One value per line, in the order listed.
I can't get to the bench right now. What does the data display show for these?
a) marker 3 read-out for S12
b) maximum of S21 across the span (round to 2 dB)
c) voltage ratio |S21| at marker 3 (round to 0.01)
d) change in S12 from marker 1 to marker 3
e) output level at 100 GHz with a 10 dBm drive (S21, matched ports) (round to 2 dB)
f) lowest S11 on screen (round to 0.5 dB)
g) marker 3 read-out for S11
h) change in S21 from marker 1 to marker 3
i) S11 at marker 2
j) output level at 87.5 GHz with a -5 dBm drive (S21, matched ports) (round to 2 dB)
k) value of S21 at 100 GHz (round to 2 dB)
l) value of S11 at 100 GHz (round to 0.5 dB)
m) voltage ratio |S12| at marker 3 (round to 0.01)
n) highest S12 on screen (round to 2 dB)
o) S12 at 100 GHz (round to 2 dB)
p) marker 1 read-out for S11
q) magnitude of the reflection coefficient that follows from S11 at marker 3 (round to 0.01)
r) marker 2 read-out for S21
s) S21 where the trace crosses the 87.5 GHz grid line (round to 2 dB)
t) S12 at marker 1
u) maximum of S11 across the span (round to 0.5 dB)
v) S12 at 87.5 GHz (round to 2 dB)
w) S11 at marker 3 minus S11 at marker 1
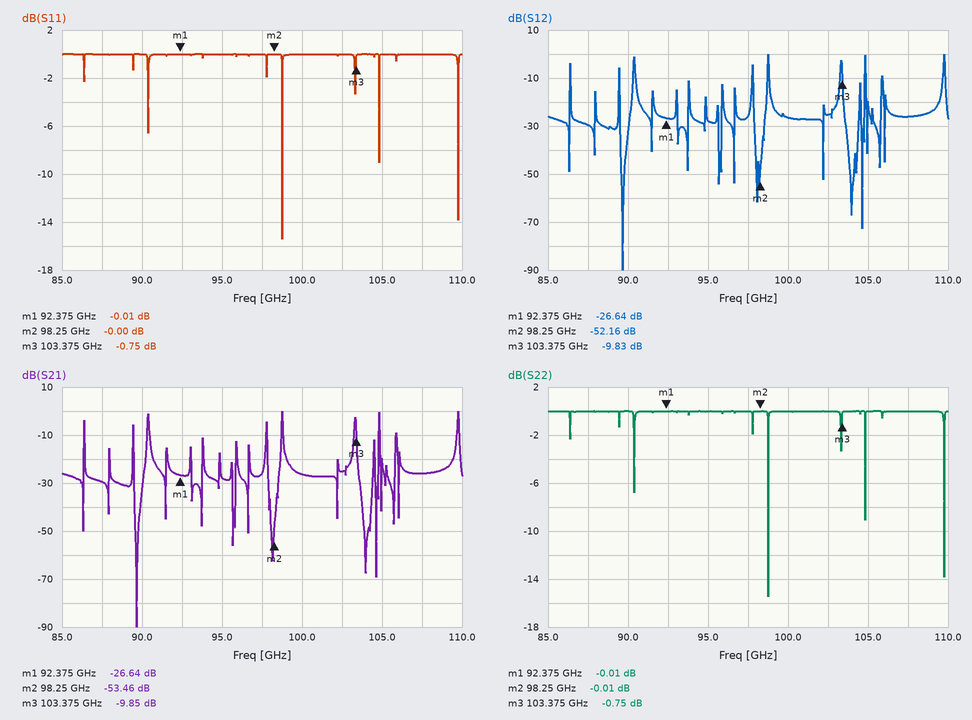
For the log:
-9.83 dB
0 dB
0.32
16.81 dB
-16 dBm
-15.5 dB
-0.75 dB
16.79 dB
-0.00 dB
-34 dBm
-26 dB
0.0 dB
0.32
0 dB
-26 dB
-0.01 dB
0.92
-53.46 dB
-30 dB
-26.64 dB
0.0 dB
-30 dB
-0.74 dB
